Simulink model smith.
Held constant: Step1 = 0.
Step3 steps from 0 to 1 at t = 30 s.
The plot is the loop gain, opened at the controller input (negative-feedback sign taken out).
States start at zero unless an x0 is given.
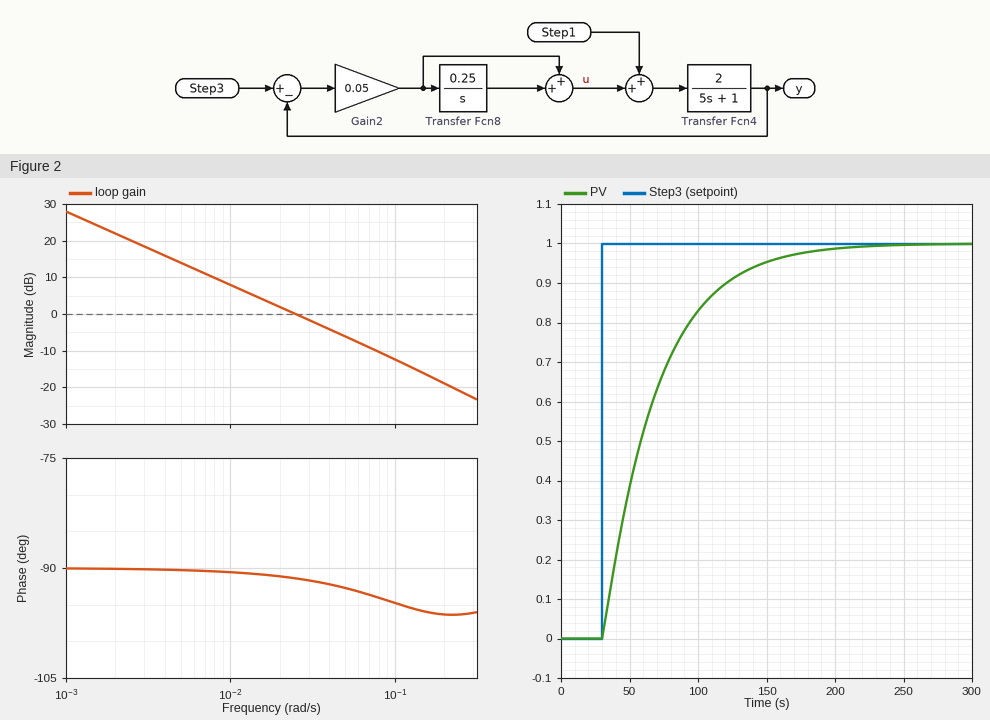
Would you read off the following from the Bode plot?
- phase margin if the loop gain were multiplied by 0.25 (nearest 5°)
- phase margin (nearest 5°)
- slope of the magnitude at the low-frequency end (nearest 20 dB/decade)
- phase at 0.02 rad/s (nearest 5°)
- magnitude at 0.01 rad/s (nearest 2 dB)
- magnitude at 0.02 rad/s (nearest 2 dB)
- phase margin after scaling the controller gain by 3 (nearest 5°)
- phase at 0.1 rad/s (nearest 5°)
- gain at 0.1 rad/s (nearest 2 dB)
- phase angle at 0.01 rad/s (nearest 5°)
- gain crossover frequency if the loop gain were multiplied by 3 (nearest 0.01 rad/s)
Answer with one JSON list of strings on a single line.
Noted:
["90°", "90°", "-20 dB/decade", "-90°", "8 dB", "2 dB", "85°", "-95°", "-12 dB", "-90°", "0.07 rad/s"]
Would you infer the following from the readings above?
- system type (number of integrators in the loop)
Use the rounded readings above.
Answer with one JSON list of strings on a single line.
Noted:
["1"]
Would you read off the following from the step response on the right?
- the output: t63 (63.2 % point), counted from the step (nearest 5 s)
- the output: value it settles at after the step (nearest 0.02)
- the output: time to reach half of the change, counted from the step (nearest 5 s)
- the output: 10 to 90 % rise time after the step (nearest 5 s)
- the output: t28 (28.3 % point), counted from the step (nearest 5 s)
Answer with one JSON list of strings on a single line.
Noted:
["40 s", "1.00", "30 s", "85 s", "15 s"]
